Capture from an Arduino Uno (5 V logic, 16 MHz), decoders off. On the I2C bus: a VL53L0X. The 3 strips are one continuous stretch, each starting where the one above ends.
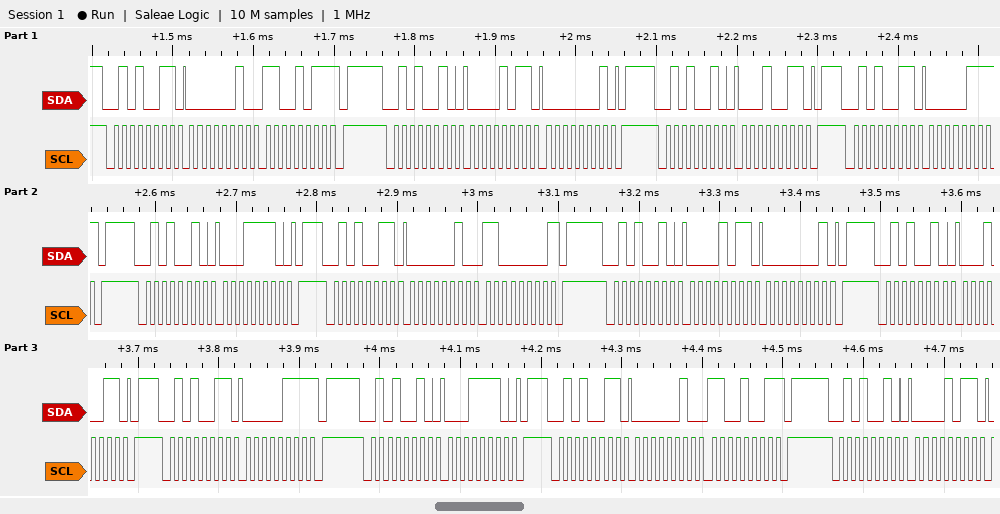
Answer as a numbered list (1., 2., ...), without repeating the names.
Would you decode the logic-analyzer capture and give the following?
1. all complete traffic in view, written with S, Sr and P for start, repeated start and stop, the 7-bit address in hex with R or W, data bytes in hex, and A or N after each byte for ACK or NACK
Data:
1. S 29R A 02 A CB N P S 29W A 0B A 01 A P S 29W A 13 A P S 29R A 07 N P S 29W A 1E A P S 29R A 02 A C0 N P S 29W A 0B A 01 A P S 29W A 13 A P S 29R A 07 N P S 29W A 1E A P S 29R A 02 A C9 N P S 29W A 0B A
